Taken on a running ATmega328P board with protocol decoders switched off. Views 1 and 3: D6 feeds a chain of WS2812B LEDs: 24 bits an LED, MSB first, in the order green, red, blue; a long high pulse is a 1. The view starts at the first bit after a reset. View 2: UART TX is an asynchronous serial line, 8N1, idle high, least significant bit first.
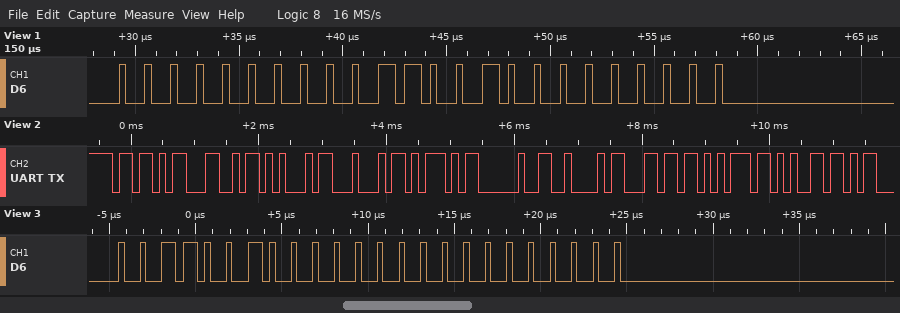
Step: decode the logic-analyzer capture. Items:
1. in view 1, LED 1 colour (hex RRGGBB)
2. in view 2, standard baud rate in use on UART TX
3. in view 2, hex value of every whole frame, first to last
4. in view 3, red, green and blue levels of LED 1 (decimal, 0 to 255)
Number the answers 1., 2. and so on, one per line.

1. #320000
2. 9600 baud
3. 5B 4C 45 44 5D 20 42 6C 75 65
4. 0, 50, 0
